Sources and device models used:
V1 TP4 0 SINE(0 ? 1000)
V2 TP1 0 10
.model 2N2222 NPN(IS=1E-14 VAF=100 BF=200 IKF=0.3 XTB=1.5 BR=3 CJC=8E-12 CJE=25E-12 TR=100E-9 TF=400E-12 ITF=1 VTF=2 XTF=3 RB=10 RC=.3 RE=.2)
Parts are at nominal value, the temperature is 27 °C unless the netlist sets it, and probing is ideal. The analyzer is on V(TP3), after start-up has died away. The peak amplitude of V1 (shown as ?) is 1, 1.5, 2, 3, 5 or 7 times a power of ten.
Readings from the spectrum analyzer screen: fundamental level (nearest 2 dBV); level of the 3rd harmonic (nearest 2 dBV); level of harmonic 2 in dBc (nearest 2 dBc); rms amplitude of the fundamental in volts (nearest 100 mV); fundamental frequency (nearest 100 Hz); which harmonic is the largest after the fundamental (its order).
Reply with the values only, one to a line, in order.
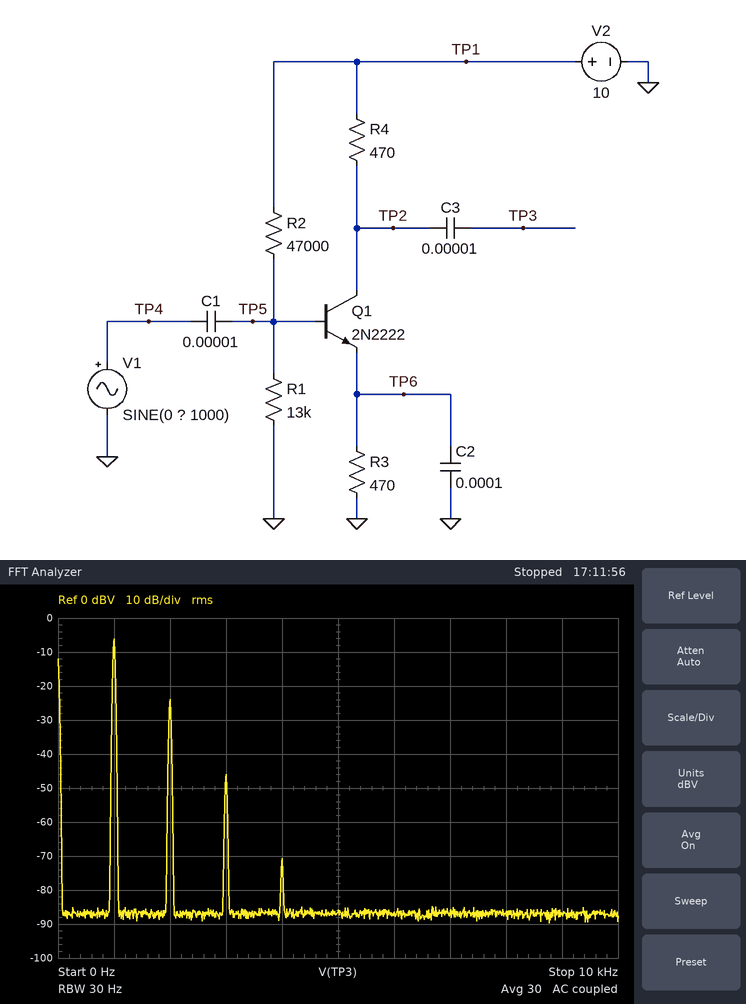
-6 dBV
-46 dBV
-18 dBc
500 mV
1.0 kHz
2
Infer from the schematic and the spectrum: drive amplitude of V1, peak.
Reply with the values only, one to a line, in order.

15 mV
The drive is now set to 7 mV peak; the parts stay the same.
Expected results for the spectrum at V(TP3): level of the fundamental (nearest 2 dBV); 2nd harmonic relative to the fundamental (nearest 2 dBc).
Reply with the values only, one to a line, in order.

-12 dBV
-24 dBc
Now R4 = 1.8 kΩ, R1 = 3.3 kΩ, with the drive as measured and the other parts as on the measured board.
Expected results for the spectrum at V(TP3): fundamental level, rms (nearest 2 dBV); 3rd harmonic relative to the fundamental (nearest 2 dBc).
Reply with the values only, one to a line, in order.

-22 dBV
-38 dBc
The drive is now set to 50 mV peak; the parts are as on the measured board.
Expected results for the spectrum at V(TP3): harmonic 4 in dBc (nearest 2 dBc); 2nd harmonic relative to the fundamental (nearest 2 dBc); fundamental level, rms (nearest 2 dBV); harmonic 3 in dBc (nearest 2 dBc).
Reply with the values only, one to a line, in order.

-34 dBc
-8 dBc
2 dBV
-20 dBc
